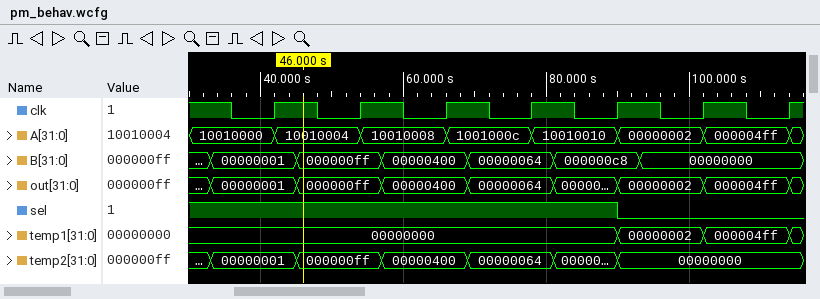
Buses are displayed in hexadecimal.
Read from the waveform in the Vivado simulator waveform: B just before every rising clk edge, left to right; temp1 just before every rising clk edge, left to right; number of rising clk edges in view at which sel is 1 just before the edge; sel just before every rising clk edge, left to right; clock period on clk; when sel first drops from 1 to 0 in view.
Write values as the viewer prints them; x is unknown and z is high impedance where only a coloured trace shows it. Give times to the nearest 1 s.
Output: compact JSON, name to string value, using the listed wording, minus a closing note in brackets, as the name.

{"B just before every rising clk edge, left to right": "00000001, 000000ff, 00000400, 00000064, 000000c8, 00000000, 00000000", "temp1 just before every rising clk edge, left to right": "00000000, 00000000, 00000000, 00000000, 00000000, 00000002, 000004ff", "number of rising clk edges in view at which sel is 1 just before the edge": "5", "sel just before every rising clk edge, left to right": "1 1 1 1 1 0 0", "clock period on clk": "12 s", "when sel first drops from 1 to 0 in view": "90 s"}
